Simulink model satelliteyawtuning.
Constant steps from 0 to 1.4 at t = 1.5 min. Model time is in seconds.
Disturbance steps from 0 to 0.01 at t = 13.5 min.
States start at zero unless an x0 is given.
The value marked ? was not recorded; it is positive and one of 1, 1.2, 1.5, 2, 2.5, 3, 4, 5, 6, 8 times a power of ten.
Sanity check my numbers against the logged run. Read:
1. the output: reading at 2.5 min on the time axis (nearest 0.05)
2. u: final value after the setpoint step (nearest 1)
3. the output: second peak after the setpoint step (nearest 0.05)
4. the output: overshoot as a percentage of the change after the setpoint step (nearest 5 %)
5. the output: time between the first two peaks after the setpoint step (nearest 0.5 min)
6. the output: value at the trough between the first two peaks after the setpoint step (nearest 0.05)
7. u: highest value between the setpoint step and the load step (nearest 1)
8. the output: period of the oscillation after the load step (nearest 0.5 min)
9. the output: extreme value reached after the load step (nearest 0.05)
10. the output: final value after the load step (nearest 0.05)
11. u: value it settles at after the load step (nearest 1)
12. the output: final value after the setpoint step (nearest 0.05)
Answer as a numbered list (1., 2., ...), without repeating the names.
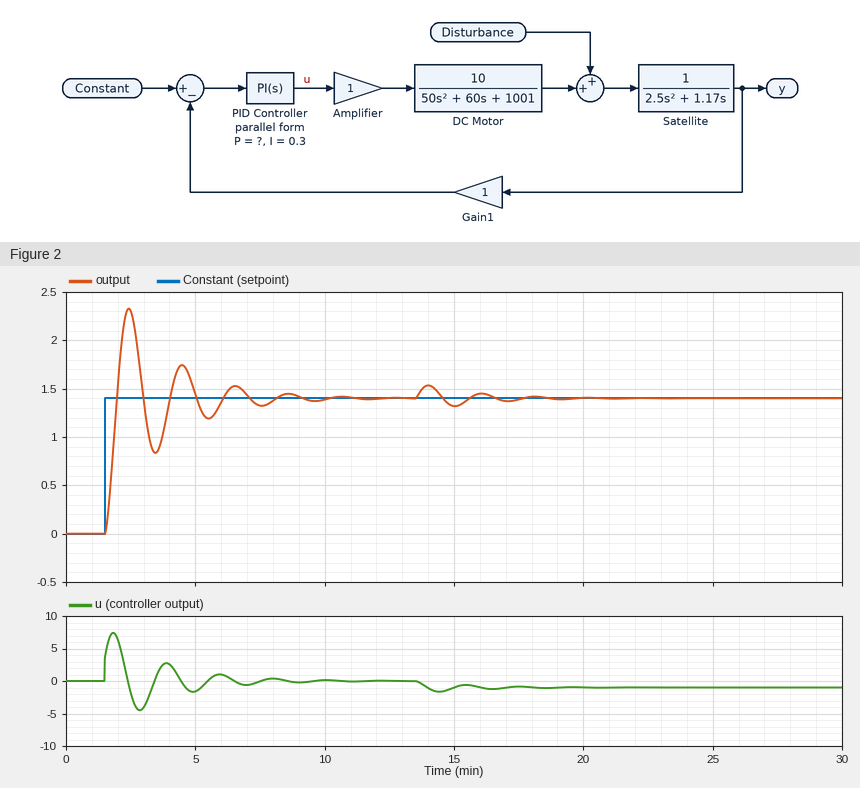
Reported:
1. 2.30
2. 0
3. 1.75
4. 65 %
5. 2.0 min
6. 0.85
7. 7
8. 2.0 min
9. 1.55
10. 1.40
11. -1
12. 1.40
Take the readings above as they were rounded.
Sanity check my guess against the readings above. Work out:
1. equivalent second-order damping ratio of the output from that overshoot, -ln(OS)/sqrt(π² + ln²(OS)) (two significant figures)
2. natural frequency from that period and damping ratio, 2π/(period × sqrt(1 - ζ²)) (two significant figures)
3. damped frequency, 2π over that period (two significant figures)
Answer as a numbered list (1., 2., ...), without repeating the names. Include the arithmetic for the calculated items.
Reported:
1. ln(0.65) = -0.431; 0.431 / sqrt(9.870 + 0.186) = 0.14
2. 2π / (2 × sqrt(1 - 0.14²)) = 3.2 rad/min
3. 2π / 2 = 3.1 rad/min
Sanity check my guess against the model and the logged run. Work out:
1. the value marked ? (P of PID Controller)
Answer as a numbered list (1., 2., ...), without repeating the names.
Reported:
1. 2.5
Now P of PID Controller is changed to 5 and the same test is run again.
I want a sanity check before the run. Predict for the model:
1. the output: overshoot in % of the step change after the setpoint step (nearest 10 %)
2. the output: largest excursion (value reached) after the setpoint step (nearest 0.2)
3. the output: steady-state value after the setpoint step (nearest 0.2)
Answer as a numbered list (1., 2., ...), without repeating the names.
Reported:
1. 40 %
2. 2.0
3. 1.4
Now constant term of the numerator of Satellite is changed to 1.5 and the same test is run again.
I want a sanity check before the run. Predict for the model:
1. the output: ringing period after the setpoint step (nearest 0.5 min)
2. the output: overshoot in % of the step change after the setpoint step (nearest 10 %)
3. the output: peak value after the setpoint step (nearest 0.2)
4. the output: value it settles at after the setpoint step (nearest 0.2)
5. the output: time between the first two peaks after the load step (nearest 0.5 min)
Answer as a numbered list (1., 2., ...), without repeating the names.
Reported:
1. 1.5 min
2. 60 %
3. 2.2
4. 1.4
5. 1.5 min
